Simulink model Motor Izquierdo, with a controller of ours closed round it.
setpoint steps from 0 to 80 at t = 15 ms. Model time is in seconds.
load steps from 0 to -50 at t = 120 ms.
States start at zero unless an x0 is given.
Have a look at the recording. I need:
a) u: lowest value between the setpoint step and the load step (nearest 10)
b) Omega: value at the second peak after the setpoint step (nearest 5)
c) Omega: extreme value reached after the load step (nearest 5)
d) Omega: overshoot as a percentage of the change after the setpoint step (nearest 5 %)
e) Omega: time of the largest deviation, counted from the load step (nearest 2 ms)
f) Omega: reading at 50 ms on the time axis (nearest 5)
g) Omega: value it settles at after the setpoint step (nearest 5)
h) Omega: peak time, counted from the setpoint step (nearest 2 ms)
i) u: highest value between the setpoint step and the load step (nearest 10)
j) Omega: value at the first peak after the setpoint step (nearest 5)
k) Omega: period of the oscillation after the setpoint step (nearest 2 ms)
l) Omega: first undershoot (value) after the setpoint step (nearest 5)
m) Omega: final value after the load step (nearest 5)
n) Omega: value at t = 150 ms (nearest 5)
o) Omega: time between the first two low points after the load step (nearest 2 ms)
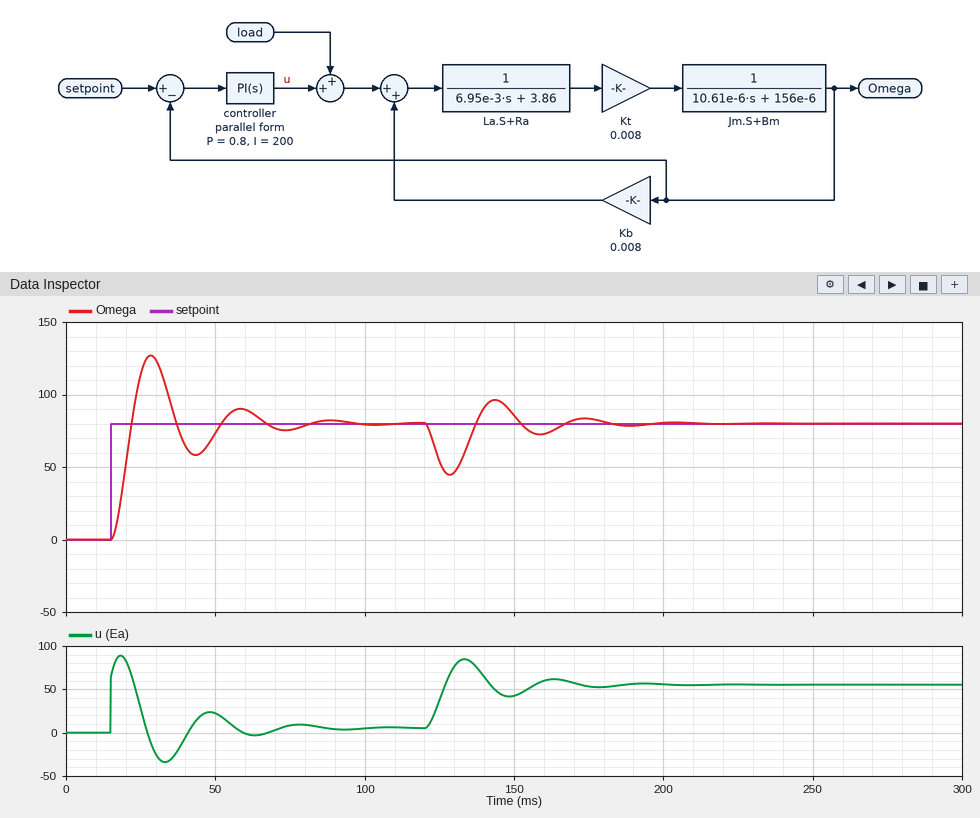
-30
90
45
60 %
8 ms
75
80
14 ms
90
125
30 ms
60
80
85
30 ms
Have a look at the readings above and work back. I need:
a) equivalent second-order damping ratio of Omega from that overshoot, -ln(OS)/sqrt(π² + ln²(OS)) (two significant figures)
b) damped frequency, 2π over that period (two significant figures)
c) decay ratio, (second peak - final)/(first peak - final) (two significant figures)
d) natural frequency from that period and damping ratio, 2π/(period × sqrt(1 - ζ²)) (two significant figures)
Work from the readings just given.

0.16
0.21 rad/ms
0.22
0.21 rad/ms
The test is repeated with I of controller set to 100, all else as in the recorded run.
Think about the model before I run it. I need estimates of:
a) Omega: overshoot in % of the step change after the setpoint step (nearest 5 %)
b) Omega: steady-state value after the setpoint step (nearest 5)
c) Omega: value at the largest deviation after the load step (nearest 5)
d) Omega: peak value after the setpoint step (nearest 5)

35 %
80
40
110
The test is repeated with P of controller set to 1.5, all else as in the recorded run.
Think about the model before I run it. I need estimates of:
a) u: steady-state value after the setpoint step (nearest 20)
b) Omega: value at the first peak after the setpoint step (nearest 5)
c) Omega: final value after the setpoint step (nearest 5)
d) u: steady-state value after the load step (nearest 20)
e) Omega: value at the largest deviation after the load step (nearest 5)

0
110
80
60
55
